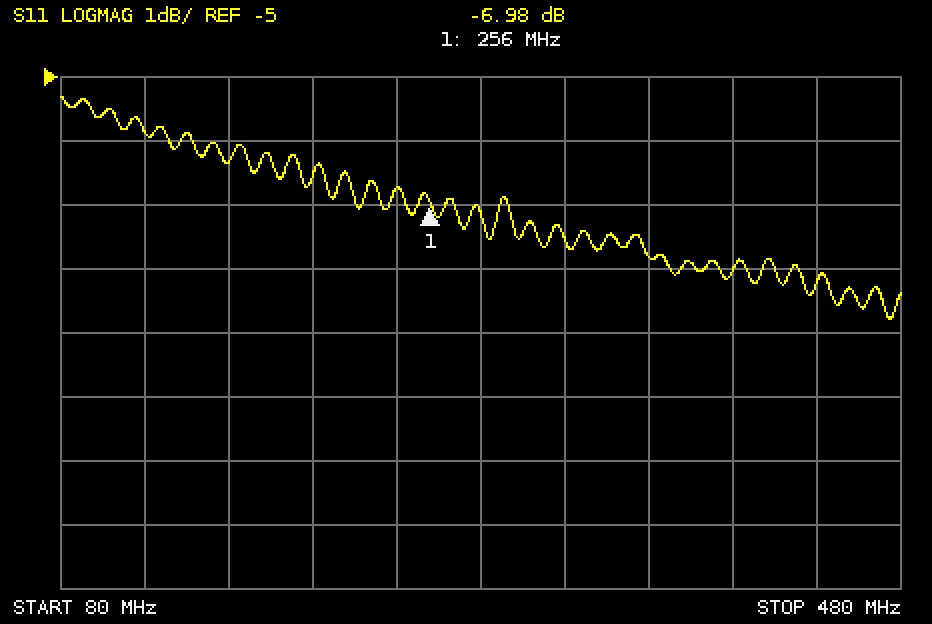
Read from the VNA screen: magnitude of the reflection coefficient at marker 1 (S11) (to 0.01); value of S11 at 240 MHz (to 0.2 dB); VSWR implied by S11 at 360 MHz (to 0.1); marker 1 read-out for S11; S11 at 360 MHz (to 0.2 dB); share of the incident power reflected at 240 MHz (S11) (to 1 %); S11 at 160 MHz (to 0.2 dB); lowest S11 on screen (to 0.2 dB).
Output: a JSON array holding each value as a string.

["0.45", "-6.8 dB", "2.4", "-6.98 dB", "-7.8 dB", "21 %", "-6.4 dB", "-8.8 dB"]
